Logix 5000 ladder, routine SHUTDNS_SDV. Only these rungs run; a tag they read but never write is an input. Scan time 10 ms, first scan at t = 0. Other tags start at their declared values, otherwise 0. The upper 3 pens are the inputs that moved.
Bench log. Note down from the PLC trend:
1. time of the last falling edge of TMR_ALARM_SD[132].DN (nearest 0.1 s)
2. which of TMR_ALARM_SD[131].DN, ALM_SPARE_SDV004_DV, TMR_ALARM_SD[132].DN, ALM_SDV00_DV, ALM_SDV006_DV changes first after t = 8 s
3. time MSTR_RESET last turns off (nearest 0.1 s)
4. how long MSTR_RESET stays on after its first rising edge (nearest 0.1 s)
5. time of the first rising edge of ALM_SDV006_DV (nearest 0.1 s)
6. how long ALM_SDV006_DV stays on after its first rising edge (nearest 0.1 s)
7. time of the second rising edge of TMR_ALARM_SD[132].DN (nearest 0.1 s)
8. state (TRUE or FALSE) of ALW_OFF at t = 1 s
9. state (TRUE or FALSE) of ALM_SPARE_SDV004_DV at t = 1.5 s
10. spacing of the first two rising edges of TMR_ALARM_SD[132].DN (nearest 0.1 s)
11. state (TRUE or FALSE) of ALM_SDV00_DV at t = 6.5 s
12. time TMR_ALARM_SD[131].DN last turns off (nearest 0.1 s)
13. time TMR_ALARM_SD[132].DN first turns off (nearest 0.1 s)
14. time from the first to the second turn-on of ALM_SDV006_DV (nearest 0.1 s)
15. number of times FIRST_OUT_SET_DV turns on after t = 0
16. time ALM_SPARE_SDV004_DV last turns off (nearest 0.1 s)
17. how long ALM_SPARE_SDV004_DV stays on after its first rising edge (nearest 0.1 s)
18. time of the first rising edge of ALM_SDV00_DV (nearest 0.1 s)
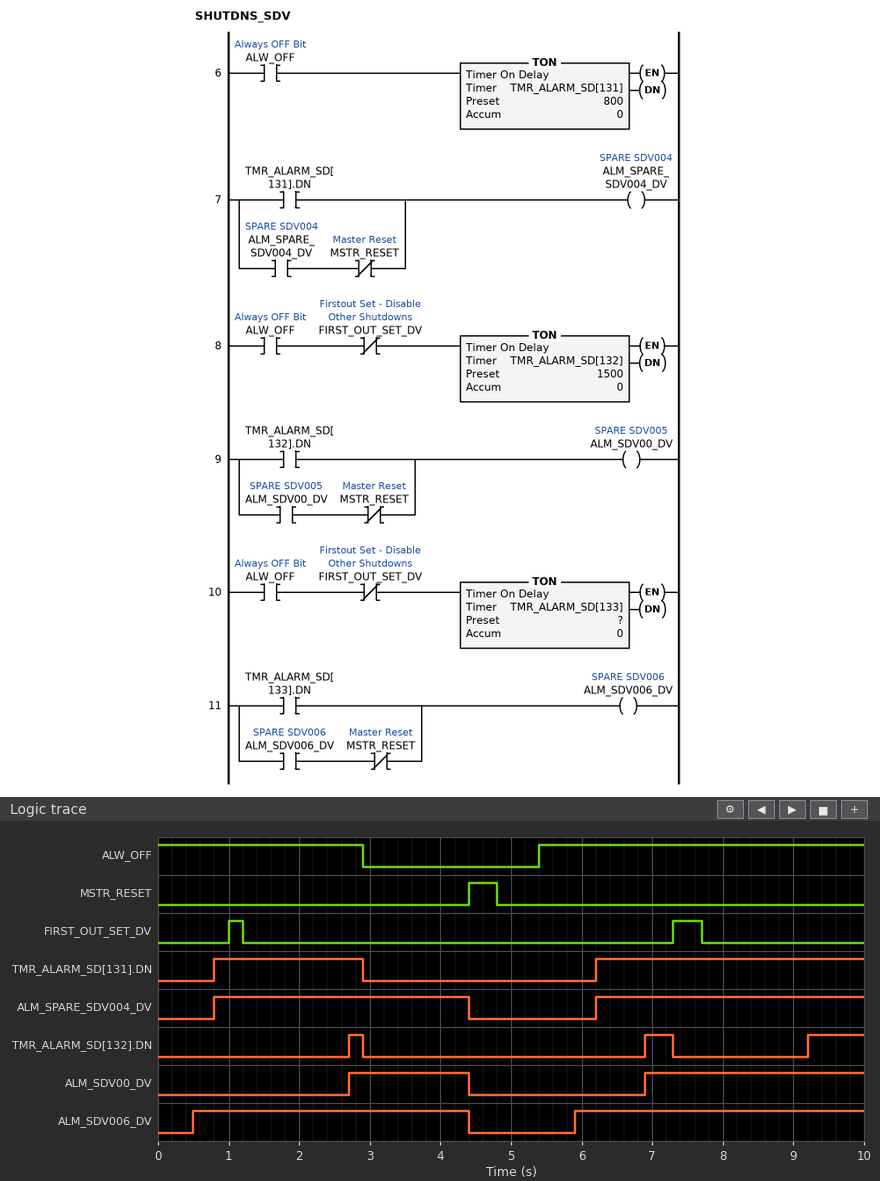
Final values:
7.3 s
TMR_ALARM_SD[132].DN
4.8 s
0.4 s
0.5 s
3.9 s
6.9 s
TRUE
TRUE
4.2 s
FALSE
2.9 s
2.9 s
5.4 s
2
4.4 s
3.6 s
2.7 s
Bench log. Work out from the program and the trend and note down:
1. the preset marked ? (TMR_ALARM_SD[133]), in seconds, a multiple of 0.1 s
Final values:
0.5 s
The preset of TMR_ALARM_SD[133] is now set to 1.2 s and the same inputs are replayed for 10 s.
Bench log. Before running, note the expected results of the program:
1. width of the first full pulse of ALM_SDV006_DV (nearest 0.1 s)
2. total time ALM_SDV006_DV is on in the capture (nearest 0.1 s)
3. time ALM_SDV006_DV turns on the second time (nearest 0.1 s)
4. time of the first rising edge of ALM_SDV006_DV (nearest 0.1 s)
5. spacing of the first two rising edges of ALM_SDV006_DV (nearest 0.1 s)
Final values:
2.0 s
5.4 s
6.6 s
2.4 s
4.2 s
